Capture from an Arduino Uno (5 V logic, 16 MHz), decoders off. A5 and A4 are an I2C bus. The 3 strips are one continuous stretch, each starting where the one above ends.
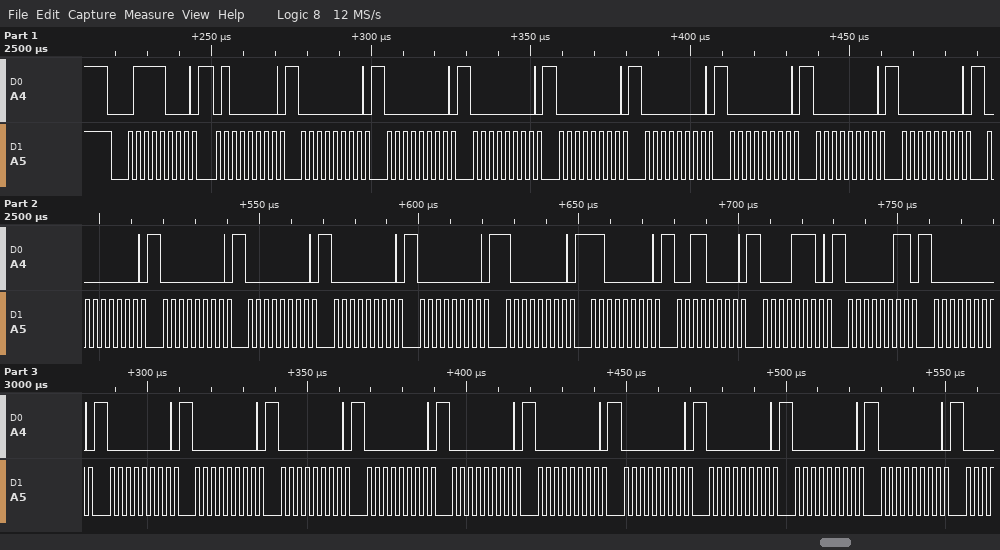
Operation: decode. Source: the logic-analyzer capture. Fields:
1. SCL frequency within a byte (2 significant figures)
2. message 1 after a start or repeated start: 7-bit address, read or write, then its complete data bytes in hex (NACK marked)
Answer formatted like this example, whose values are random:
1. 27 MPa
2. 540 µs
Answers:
1. 400 kHz
2. 0x3C write: 40 00 00 00 00 00 00 00 00 00 00 00 00 00 80 C0 30 0E 03 00 00 00 00 00 00 00 00 00 00 00
